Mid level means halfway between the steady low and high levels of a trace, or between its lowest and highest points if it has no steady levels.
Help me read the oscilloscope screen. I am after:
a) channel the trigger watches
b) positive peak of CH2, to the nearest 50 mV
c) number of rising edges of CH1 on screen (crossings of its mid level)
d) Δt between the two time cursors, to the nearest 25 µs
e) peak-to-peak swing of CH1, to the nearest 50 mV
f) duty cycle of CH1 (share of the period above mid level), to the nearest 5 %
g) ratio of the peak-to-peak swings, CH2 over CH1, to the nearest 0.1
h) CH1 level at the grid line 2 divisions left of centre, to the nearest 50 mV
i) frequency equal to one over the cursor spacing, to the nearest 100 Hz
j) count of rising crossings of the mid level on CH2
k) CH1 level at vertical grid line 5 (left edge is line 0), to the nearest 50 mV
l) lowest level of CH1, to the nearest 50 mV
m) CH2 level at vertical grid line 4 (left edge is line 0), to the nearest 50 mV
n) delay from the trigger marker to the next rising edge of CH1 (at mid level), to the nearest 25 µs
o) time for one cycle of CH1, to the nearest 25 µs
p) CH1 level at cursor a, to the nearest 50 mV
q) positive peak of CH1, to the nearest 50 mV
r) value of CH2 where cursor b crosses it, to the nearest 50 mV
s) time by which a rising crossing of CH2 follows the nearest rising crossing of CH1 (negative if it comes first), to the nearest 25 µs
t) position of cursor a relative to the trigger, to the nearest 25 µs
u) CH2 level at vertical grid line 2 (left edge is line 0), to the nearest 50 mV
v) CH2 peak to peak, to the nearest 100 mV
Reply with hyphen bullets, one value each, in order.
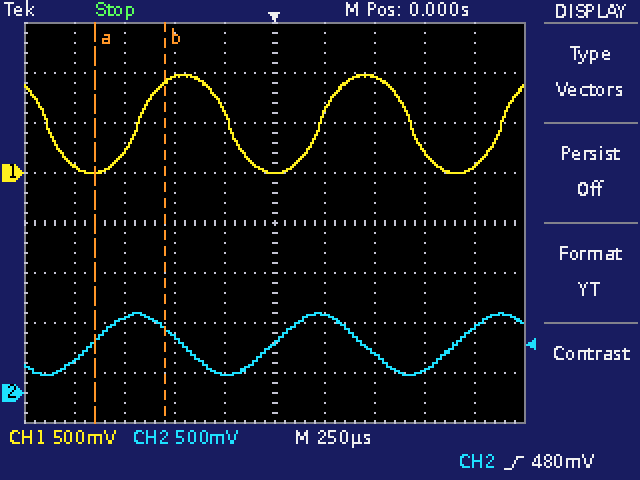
- CH2
- 800 mV
- 3
- 350 µs
- 1.00 V
- 50 %
- 0.6
- 950 mV
- 2.9 kHz
- 3
- 0 mV
- 0 mV
- 200 mV
- 225 µs
- 900 µs
- 0 mV
- 1.00 V
- 650 mV
- -225 µs
- -900 µs
- 750 mV
- 600 mV
